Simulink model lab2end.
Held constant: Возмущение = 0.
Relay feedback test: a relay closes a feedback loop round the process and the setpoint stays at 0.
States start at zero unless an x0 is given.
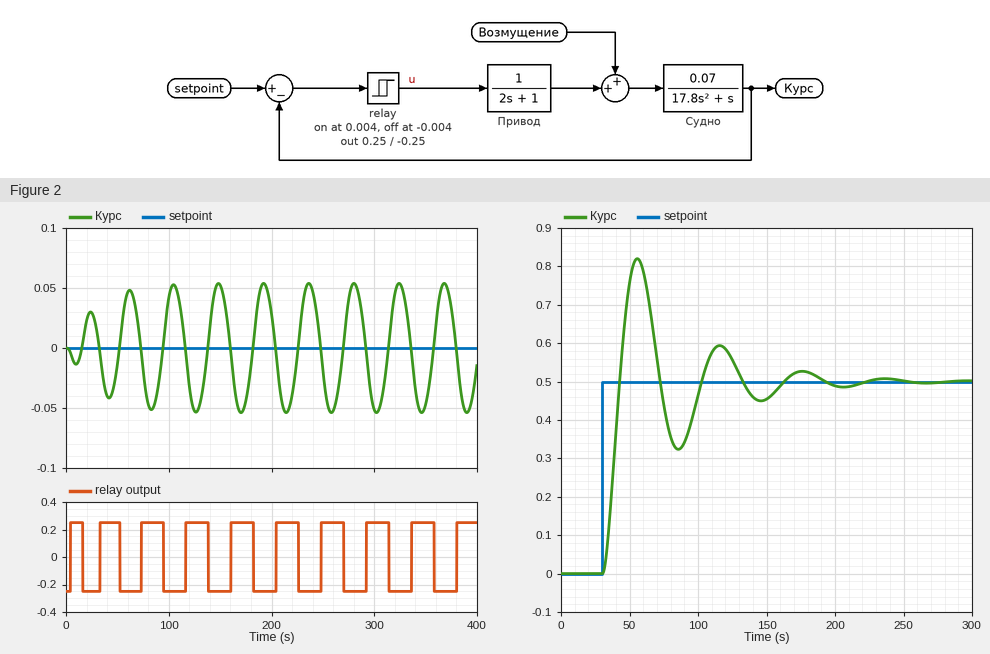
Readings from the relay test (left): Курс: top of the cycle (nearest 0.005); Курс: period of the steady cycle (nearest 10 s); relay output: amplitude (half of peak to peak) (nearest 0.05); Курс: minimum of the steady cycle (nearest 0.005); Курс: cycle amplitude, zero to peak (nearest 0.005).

0.055
40 s
0.25
-0.055
0.055
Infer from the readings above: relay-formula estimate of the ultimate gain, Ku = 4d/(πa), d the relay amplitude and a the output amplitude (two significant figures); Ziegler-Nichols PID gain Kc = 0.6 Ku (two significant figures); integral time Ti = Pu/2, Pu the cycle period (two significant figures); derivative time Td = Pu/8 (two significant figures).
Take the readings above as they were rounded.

5.8
3.5
20 s
5.0 s
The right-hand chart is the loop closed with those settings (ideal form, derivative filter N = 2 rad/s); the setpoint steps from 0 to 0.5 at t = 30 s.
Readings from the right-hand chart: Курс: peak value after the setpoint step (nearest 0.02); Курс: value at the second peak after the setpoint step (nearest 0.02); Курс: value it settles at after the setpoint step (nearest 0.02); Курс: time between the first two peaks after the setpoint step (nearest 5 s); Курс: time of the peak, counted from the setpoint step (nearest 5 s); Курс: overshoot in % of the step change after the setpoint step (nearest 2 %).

0.82
0.60
0.50
60 s
25 s
64 %
